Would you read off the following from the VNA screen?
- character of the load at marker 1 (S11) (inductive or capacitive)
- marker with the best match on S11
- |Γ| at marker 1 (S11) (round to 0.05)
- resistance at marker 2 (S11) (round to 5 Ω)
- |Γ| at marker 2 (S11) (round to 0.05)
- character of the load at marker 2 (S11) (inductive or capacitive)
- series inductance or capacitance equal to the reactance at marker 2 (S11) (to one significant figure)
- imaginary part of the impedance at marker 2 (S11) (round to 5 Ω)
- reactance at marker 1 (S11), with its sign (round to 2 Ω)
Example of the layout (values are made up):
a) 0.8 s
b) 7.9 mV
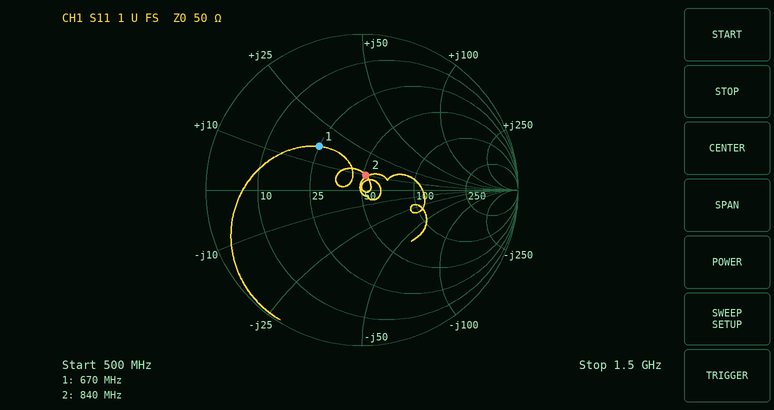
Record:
a) inductive
b) marker 2
c) 0.40
d) 50 Ω
e) 0.10
f) inductive
g) 2 nH
h) +10 Ω
i) +16 Ω
